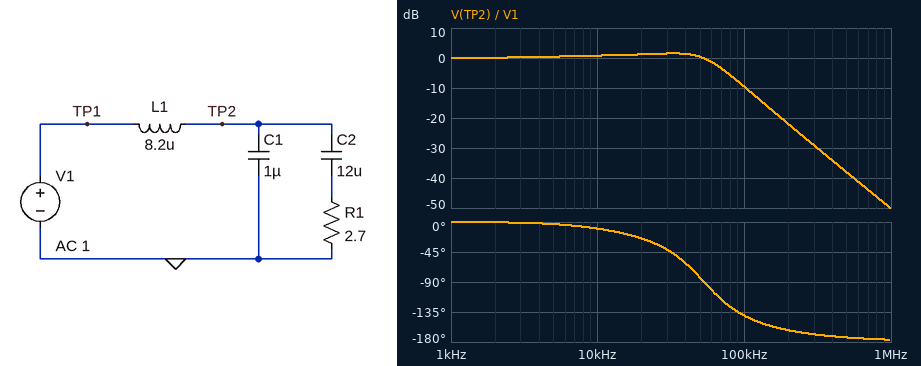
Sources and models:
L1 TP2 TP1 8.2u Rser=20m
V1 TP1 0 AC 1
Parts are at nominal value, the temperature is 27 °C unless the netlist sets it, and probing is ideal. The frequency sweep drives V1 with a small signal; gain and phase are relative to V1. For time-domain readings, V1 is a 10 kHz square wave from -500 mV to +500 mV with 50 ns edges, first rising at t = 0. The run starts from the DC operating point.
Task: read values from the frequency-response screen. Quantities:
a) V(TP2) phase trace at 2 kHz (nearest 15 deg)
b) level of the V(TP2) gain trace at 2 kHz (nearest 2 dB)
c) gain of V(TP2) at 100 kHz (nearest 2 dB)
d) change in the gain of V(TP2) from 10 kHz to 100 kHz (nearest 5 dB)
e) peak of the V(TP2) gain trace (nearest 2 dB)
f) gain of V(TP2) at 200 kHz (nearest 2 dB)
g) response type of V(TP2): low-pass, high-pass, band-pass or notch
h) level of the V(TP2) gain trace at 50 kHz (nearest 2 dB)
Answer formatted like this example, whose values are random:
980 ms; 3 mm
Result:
0 deg; 0 dB; -10 dB; -10 dB; 2 dB; -22 dB; low-pass; 0 dB
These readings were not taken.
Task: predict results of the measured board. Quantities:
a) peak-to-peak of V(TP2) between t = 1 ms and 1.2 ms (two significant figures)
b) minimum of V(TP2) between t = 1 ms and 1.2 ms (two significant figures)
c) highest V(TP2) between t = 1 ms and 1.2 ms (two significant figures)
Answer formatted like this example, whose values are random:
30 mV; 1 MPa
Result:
1.4 V; -700 mV; 700 mV
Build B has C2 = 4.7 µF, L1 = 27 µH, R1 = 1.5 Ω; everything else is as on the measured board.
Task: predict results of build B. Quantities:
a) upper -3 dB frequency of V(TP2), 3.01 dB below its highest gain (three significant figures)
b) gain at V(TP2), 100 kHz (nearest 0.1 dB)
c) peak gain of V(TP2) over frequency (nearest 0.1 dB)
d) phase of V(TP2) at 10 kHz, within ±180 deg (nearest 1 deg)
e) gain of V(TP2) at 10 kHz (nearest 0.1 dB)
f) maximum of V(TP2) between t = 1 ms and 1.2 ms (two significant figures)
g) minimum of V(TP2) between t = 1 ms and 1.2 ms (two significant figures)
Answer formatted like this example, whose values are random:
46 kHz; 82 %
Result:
15.6 kHz; -24.2 dB; 7.7 dB; -22 deg; 5.8 dB; 1.2 V; -1.2 V
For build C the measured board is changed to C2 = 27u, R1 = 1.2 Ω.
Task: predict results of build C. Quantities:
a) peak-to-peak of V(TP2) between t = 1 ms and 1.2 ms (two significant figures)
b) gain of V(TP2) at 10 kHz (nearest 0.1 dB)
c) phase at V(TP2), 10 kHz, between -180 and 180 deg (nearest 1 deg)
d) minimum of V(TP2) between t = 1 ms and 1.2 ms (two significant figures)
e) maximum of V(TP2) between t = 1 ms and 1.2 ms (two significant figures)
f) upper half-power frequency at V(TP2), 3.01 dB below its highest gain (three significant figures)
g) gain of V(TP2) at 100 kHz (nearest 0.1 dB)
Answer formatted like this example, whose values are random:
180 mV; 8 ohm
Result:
1.2 V; 1.1 dB; -24 deg; -610 mV; 610 mV; 26.1 kHz; -13.9 dB
